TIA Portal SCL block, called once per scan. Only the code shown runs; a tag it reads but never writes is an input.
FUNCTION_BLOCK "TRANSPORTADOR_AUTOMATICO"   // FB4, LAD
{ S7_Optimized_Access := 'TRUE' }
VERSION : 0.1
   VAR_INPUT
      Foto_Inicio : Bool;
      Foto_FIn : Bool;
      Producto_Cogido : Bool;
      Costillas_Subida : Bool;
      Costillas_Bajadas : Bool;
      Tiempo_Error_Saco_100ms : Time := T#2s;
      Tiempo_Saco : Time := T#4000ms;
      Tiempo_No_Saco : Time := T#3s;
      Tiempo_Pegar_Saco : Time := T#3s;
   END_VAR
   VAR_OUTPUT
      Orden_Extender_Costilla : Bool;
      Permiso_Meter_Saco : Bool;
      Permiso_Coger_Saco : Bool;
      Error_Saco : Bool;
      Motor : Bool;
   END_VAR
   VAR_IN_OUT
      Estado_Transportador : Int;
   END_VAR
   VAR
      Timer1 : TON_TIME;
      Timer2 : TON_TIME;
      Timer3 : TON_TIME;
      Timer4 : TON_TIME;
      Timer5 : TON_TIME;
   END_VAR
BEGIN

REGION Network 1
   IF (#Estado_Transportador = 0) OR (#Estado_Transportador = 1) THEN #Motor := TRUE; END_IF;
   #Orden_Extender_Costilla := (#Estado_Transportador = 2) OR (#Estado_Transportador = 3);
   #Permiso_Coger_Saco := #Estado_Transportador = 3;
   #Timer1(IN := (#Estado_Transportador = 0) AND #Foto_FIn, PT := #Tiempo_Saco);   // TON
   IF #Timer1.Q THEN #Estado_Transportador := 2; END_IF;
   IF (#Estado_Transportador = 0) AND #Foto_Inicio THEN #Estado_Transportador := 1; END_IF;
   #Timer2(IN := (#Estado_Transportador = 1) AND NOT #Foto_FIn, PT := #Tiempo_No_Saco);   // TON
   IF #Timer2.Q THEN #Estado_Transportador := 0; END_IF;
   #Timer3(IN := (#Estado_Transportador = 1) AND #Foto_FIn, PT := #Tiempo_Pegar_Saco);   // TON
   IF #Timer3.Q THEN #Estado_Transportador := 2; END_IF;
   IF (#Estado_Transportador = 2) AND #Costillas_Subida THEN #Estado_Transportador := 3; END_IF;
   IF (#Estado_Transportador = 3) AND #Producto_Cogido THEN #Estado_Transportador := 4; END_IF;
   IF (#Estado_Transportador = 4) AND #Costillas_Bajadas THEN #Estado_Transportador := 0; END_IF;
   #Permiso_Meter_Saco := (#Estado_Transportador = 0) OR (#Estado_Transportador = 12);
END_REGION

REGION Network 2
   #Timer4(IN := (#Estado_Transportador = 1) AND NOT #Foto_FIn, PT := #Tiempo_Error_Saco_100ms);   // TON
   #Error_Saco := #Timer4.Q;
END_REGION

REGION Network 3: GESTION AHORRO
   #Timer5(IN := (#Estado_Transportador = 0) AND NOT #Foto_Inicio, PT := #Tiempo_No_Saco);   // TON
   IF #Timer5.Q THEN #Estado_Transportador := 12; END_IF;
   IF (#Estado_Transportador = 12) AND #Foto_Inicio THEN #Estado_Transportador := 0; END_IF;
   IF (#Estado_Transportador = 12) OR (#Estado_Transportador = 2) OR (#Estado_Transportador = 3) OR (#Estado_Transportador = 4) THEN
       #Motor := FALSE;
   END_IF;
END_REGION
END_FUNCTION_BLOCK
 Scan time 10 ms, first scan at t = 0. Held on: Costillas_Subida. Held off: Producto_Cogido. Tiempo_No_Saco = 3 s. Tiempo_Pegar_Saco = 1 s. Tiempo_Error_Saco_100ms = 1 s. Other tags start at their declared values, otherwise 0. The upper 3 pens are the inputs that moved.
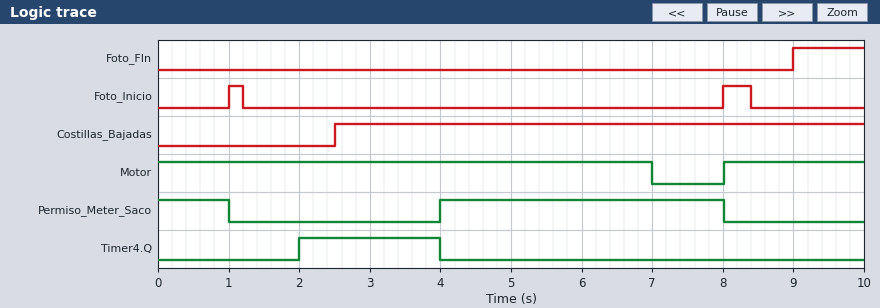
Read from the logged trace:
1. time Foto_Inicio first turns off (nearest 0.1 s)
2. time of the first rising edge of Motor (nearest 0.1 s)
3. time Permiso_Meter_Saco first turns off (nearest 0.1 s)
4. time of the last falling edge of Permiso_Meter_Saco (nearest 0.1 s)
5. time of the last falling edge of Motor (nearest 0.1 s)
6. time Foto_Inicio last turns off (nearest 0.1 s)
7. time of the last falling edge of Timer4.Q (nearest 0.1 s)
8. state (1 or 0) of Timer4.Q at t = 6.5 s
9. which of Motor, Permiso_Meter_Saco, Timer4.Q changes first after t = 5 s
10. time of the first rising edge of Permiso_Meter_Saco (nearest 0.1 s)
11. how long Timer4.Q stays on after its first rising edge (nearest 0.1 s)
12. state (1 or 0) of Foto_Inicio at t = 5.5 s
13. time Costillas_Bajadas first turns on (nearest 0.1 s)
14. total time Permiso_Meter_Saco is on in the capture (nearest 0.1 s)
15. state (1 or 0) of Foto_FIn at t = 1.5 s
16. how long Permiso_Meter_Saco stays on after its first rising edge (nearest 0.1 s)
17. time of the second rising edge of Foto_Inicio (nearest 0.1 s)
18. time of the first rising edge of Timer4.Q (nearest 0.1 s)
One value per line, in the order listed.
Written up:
1.2 s
8.0 s
1.0 s
8.0 s
7.0 s
8.4 s
4.0 s
0
Motor
4.0 s
2.0 s
0
2.5 s
5.0 s
0
4.0 s
8.0 s
2.0 s
